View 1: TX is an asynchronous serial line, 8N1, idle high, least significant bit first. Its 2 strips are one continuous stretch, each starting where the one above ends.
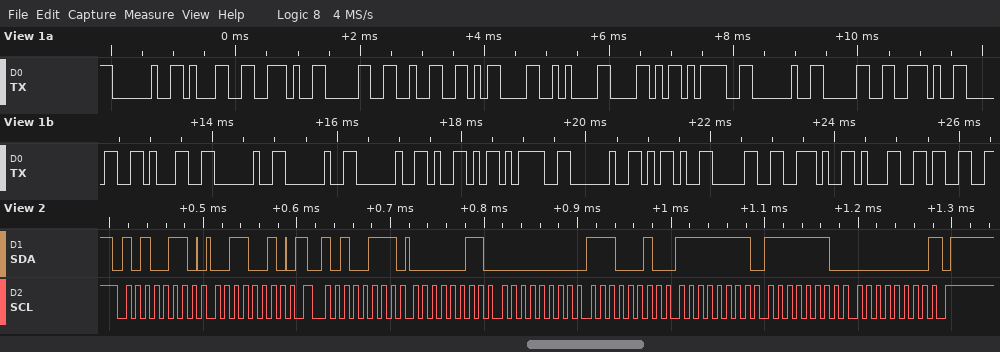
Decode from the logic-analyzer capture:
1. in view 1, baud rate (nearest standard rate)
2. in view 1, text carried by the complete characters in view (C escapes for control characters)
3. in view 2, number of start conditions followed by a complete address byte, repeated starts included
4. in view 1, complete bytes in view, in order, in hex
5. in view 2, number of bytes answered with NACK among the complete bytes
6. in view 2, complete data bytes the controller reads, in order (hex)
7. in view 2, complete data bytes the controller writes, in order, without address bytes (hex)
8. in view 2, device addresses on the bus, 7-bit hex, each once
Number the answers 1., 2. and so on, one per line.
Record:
1. 9600 baud
2. " 1.02\r\nX= 0.01   Y= -0.13"
3. 2
4. 0x20 0x31 0x2E 0x30 0x32 0x0D 0x0A 0x58 0x3D 0x20 0x30 0x2E 0x30 0x31 0x20 0x20 0x20 0x59 0x3D 0x20 0x2D 0x30 0x2E 0x31 0x33
5. 1
6. 03 00 E2 FF FE 00
7. 32
8. 0x53
